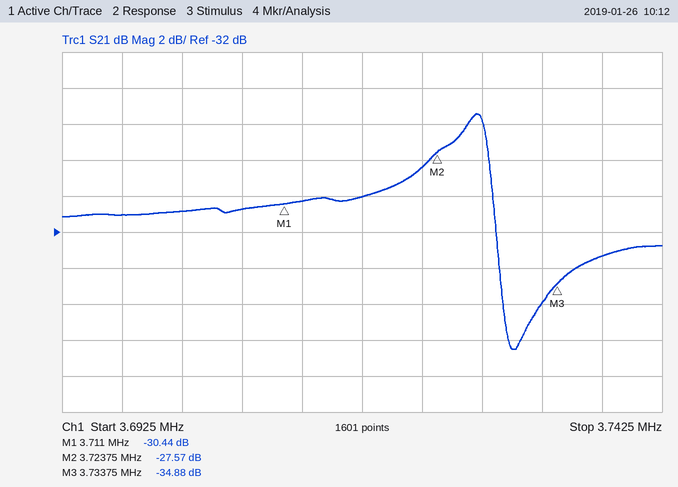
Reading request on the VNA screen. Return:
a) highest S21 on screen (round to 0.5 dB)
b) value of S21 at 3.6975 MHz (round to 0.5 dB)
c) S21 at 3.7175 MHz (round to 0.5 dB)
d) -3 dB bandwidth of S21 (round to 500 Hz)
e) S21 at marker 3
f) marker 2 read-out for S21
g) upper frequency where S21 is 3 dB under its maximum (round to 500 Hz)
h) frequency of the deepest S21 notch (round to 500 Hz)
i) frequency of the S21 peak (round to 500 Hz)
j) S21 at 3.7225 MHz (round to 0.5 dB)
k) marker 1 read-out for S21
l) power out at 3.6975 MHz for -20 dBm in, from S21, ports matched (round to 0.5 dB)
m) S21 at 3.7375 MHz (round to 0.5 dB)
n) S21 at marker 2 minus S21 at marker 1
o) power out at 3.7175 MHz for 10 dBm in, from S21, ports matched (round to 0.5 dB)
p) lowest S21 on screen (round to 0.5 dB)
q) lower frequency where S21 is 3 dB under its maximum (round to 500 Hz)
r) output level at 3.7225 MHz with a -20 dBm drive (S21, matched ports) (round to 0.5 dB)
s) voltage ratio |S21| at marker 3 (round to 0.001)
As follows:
-25.5 dB
-31.0 dB
-30.0 dB
5.5 kHz
-34.88 dB
-27.57 dB
3.7280 MHz
3.7300 MHz
3.7270 MHz
-28.5 dB
-30.44 dB
-51.0 dBm
-33.5 dB
2.87 dB
-20.0 dBm
-38.5 dB
3.7225 MHz
-48.5 dBm
0.018
